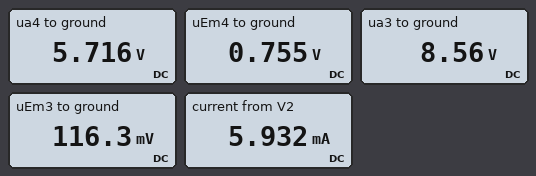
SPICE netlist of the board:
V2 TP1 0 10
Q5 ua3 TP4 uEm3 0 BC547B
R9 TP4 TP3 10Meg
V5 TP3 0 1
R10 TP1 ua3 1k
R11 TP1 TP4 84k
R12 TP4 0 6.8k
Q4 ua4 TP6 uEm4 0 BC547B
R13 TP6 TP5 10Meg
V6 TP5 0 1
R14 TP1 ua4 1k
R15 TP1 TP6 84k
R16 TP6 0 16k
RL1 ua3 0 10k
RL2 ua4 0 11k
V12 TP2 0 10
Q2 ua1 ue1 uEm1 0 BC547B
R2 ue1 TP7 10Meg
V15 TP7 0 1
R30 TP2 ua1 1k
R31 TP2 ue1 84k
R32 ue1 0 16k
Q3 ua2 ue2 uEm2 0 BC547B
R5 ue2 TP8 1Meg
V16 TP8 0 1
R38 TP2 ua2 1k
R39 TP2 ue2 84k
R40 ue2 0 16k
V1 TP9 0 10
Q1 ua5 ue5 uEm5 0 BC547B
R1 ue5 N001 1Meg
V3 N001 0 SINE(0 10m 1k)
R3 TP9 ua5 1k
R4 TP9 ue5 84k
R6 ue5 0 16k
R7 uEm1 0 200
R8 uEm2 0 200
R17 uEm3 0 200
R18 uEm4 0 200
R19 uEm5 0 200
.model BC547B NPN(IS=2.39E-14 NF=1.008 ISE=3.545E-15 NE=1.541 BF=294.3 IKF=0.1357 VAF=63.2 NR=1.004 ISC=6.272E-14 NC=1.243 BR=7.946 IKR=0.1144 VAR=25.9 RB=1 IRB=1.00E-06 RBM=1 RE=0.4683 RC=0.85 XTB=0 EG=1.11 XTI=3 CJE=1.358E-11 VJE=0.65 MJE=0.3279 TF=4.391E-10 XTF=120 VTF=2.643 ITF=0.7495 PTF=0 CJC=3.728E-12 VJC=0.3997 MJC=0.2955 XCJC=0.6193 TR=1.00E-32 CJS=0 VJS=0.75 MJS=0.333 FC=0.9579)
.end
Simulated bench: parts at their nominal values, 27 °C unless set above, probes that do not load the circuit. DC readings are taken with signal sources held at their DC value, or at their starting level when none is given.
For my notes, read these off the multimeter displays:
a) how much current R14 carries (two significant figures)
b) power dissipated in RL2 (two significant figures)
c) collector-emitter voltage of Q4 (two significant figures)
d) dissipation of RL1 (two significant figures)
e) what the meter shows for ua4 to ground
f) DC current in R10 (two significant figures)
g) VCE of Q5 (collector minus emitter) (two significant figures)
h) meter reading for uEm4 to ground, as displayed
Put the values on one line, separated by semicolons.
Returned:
4.3 mA; 3.0 mW; 5.0 V; 7.3 mW; 5.716 V; 1.4 mA; 8.4 V; 0.755 V
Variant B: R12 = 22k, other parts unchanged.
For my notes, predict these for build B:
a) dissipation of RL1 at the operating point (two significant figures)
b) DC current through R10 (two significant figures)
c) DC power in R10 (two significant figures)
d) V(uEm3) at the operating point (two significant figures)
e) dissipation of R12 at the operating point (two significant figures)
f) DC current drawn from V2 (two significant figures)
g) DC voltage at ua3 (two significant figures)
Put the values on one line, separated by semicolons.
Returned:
1.8 mW; 5.7 mA; 33 mW; 1.1 V; 140 µW; 10 mA; 4.3 V
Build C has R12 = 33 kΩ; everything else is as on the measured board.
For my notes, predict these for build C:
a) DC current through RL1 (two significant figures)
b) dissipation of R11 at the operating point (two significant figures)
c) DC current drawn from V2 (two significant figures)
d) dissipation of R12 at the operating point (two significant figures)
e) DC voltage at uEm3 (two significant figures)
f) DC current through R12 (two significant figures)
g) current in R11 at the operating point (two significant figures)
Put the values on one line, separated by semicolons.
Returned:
240 µA; 730 µW; 12 mA; 140 µW; 1.5 V; 66 µA; 93 µA
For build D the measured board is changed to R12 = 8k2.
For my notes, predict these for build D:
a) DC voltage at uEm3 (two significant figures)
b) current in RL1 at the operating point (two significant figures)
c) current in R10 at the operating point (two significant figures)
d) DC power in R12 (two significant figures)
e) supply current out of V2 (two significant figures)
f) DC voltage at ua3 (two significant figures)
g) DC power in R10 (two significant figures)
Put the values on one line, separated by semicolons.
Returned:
220 mV; 810 µA; 1.9 mA; 91 µW; 6.4 mA; 8.1 V; 3.7 mW
